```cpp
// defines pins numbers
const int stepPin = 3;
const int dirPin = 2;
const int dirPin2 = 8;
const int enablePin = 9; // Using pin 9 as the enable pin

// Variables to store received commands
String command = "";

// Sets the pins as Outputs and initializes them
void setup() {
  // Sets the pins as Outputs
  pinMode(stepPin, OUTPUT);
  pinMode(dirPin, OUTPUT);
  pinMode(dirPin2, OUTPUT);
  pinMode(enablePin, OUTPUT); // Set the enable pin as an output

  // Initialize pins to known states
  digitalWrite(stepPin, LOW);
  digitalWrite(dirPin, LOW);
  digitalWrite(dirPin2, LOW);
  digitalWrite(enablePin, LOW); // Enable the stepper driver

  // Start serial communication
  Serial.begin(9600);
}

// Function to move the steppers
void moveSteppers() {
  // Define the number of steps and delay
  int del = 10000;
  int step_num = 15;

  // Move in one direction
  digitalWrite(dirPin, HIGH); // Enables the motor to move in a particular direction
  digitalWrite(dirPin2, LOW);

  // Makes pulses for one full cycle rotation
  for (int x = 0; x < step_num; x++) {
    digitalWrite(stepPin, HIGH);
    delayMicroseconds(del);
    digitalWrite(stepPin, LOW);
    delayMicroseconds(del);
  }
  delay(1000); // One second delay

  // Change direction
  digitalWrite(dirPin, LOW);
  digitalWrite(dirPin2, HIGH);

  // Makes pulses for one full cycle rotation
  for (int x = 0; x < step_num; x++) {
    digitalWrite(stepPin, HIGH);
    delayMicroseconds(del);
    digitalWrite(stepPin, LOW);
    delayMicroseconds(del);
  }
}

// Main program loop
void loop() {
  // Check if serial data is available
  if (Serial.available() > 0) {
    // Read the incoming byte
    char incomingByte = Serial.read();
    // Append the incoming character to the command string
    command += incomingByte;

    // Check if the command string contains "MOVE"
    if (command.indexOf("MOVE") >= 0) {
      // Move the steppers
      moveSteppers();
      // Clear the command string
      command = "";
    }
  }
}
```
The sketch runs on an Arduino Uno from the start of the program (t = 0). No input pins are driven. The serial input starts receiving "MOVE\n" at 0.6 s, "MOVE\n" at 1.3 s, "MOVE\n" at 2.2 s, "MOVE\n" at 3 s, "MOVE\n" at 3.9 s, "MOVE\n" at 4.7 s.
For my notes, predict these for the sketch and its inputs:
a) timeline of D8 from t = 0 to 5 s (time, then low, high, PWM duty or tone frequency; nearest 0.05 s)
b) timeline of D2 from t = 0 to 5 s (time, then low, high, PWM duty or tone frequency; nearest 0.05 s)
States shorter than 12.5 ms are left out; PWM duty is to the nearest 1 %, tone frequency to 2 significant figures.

0 s low; 1.9 s high; 2.2 s low; 3.5 s high; 3.8 s low
0 s low; 0.6 s high; 1.9 s low; 2.2 s high; 3.5 s low; 3.8 s high
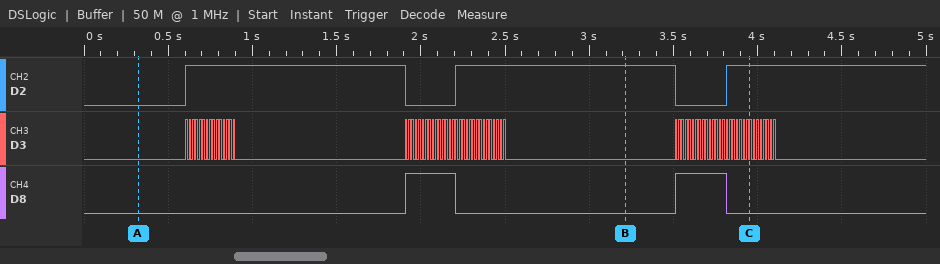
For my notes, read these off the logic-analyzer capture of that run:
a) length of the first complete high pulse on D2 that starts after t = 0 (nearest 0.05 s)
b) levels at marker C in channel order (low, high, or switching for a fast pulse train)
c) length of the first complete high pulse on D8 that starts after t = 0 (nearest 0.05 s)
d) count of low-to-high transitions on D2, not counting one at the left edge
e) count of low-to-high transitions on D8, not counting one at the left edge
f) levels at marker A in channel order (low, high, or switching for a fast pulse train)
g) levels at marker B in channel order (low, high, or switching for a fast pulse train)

1.30 s
D2 high, D3 switching, D8 low
0.30 s
3
2
D2 low, D3 low, D8 low
D2 high, D3 low, D8 low
